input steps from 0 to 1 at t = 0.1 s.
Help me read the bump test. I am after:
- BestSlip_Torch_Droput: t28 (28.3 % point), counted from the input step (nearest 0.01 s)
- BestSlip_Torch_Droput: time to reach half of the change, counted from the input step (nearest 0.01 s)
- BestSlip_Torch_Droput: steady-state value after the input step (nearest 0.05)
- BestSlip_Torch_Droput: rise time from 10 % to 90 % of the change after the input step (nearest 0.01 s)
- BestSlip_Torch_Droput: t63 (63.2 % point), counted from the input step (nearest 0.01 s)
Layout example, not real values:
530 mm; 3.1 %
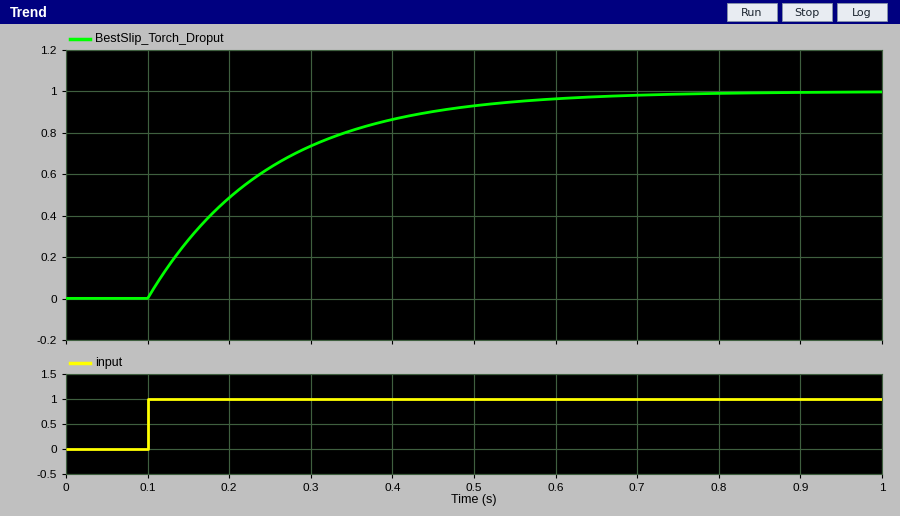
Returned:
0.05 s; 0.10 s; 1.00; 0.33 s; 0.15 s
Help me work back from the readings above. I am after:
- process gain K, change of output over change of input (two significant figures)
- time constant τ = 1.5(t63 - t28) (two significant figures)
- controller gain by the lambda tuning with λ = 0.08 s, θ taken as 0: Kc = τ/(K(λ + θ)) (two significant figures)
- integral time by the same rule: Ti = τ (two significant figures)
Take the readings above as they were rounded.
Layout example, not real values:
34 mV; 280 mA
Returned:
1.0; 0.15 s; 1.9; 0.15 s
